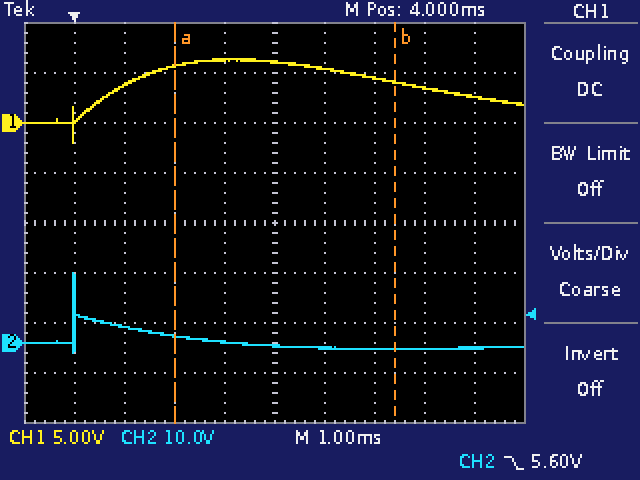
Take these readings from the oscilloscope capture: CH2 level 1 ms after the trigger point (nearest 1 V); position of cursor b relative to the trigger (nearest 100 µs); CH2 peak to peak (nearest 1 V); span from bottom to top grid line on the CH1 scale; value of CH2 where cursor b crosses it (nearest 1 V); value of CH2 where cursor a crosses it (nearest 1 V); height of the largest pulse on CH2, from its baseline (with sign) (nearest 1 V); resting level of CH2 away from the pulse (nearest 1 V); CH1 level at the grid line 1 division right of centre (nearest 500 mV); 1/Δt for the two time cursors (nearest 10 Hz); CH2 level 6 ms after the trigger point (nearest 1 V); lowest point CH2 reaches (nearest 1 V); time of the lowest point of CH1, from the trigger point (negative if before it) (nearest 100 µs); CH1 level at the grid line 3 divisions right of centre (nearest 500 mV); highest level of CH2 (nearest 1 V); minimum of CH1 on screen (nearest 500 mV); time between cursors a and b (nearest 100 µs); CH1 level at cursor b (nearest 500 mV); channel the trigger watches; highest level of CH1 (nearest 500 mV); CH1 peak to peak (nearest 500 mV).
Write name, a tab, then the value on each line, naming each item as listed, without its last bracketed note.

CH2 level 1 ms after the trigger point	3 V
position of cursor b relative to the trigger	+6.4 ms
CH2 peak to peak	16 V
span from bottom to top grid line on the CH1 scale	40 V
value of CH2 where cursor b crosses it	-1 V
value of CH2 where cursor a crosses it	1 V
height of the largest pulse on CH2, from its baseline (with sign)	+15 V
resting level of CH2 away from the pulse	-1 V
CH1 level at the grid line 1 division right of centre	5.5 V
1/Δt for the two time cursors	230 Hz
CH2 level 6 ms after the trigger point	-1 V
lowest point CH2 reaches	-2 V
time of the lowest point of CH1, from the trigger point (negative if before it)	0.0 ms
CH1 level at the grid line 3 divisions right of centre	3.5 V
highest level of CH2	14 V
minimum of CH1 on screen	-2.0 V
time between cursors a and b	4.4 ms
CH1 level at cursor b	4.0 V
channel the trigger watches	CH2
highest level of CH1	6.5 V
CH1 peak to peak	8.5 V
